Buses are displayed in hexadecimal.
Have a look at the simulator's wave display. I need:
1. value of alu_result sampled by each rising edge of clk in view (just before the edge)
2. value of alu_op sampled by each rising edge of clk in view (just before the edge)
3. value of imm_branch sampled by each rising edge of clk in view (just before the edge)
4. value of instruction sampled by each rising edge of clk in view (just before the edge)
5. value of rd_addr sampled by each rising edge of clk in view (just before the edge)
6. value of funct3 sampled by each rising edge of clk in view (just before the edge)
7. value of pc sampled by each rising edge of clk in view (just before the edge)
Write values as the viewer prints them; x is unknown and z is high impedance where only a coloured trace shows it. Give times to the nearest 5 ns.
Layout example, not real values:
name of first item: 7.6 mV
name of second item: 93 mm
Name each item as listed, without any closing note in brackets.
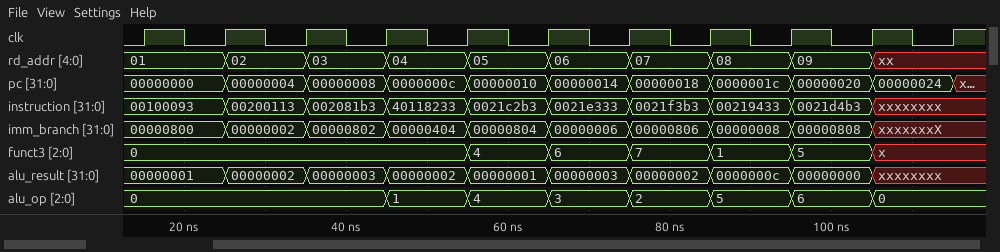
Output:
value of alu_result sampled by each rising edge of clk in view: 00000001, 00000001, 00000002, 00000003, 00000002, 00000001, 00000003, 00000002, 0000000c, 00000000, xxxxxxxx
value of alu_op sampled by each rising edge of clk in view: 0, 0, 0, 0, 1, 4, 3, 2, 5, 6, 0
value of imm_branch sampled by each rising edge of clk in view: 00000800, 00000800, 00000002, 00000802, 00000404, 00000804, 00000006, 00000806, 00000008, 00000808, xxxxxxxX
value of instruction sampled by each rising edge of clk in view: 00100093, 00100093, 00200113, 002081b3, 40118233, 0021c2b3, 0021e333, 0021f3b3, 00219433, 0021d4b3, xxxxxxxx
value of rd_addr sampled by each rising edge of clk in view: 01, 01, 02, 03, 04, 05, 06, 07, 08, 09, xx
value of funct3 sampled by each rising edge of clk in view: 0, 0, 0, 0, 0, 4, 6, 7, 1, 5, x
value of pc sampled by each rising edge of clk in view: 00000000, 00000000, 00000004, 00000008, 0000000c, 00000010, 00000014, 00000018, 0000001c, 00000020, 00000024
